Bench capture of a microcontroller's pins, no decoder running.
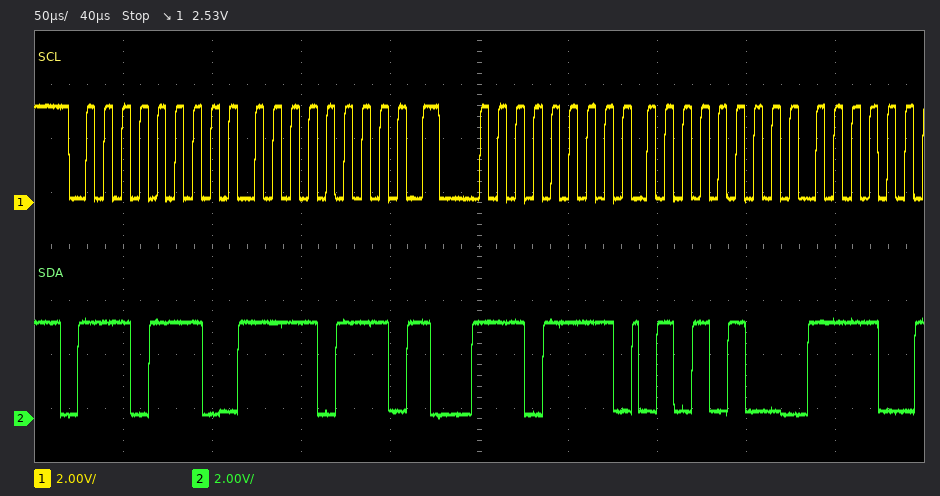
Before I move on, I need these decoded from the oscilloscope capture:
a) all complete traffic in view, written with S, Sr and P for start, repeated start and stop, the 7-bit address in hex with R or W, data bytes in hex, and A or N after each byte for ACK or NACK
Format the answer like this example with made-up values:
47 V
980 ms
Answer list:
S 77W A F7 A Sr 77R A 54 A
